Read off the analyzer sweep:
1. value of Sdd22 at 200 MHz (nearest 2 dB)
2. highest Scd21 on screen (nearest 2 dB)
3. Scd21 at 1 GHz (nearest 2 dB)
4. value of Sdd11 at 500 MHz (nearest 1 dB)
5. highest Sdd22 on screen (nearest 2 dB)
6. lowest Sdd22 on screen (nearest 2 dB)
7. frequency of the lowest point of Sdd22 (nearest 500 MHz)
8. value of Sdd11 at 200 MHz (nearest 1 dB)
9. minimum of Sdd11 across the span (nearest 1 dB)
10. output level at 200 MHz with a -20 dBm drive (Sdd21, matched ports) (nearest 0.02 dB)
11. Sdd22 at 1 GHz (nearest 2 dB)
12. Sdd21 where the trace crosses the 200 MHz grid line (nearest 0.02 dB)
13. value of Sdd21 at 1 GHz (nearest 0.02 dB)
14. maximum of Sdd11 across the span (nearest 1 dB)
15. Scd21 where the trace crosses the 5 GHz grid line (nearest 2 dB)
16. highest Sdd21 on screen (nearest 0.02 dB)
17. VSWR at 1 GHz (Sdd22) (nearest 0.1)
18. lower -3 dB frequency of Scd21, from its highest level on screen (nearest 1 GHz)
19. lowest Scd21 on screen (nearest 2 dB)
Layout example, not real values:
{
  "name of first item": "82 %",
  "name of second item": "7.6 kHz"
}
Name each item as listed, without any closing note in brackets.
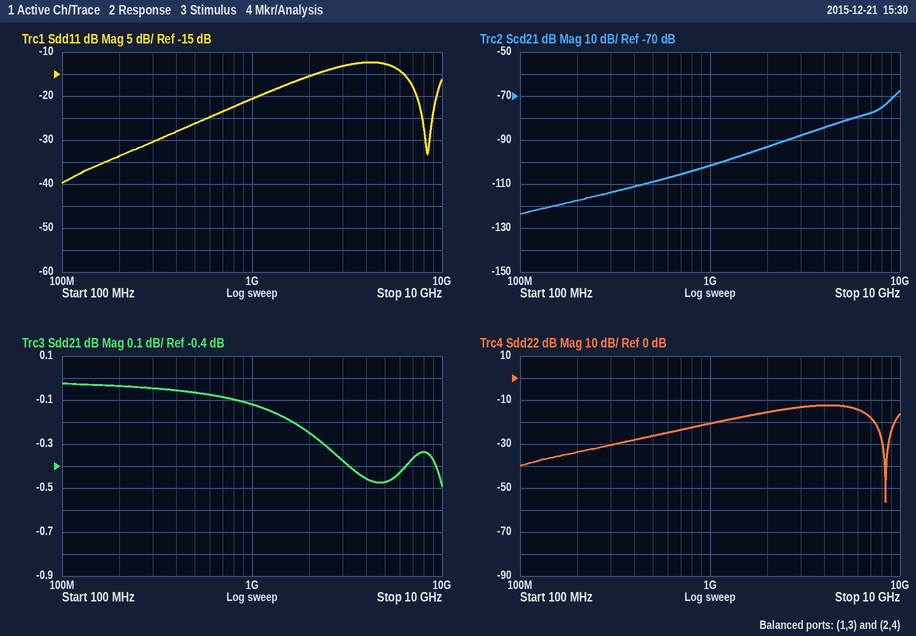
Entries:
{
  "value of Sdd22 at 200 MHz": "-34 dB",
  "highest Scd21 on screen": "-68 dB",
  "Scd21 at 1 GHz": "-102 dB",
  "value of Sdd11 at 500 MHz": "-26 dB",
  "highest Sdd22 on screen": "-12 dB",
  "lowest Sdd22 on screen": "-56 dB",
  "frequency of the lowest point of Sdd22": "8.5 GHz",
  "value of Sdd11 at 200 MHz": "-34 dB",
  "minimum of Sdd11 across the span": "-40 dB",
  "output level at 200 MHz with a -20 dBm drive (Sdd21, matched ports)": "-20.04 dBm",
  "Sdd22 at 1 GHz": "-20 dB",
  "Sdd21 where the trace crosses the 200 MHz grid line": "-0.04 dB",
  "value of Sdd21 at 1 GHz": "-0.12 dB",
  "maximum of Sdd11 across the span": "-12 dB",
  "Scd21 where the trace crosses the 5 GHz grid line": "-82 dB",
  "highest Sdd21 on screen": "-0.02 dB",
  "VSWR at 1 GHz (Sdd22)": "1.2",
  "lower -3 dB frequency of Scd21, from its highest level on screen": "9 GHz",
  "lowest Scd21 on screen": "-124 dB"
}
